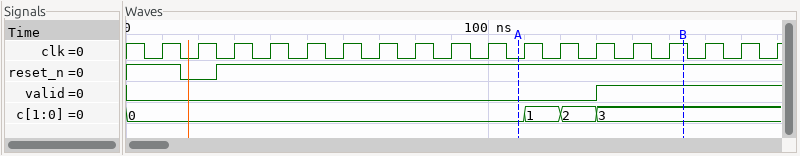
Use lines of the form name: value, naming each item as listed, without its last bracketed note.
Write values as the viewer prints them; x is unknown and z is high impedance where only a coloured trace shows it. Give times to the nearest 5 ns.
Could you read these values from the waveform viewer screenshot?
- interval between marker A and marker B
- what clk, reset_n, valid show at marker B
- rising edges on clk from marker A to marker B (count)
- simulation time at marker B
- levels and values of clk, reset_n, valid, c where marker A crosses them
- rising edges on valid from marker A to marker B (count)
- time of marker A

interval between marker A and marker B: 45 ns
what clk, reset_n, valid show at marker B: clk=1, reset_n=1, valid=1
rising edges on clk from marker A to marker B: 5
simulation time at marker B: 155 ns
levels and values of clk, reset_n, valid, c where marker A crosses them: clk=0, reset_n=1, valid=0, c=0
rising edges on valid from marker A to marker B: 1
time of marker A: 110 ns
